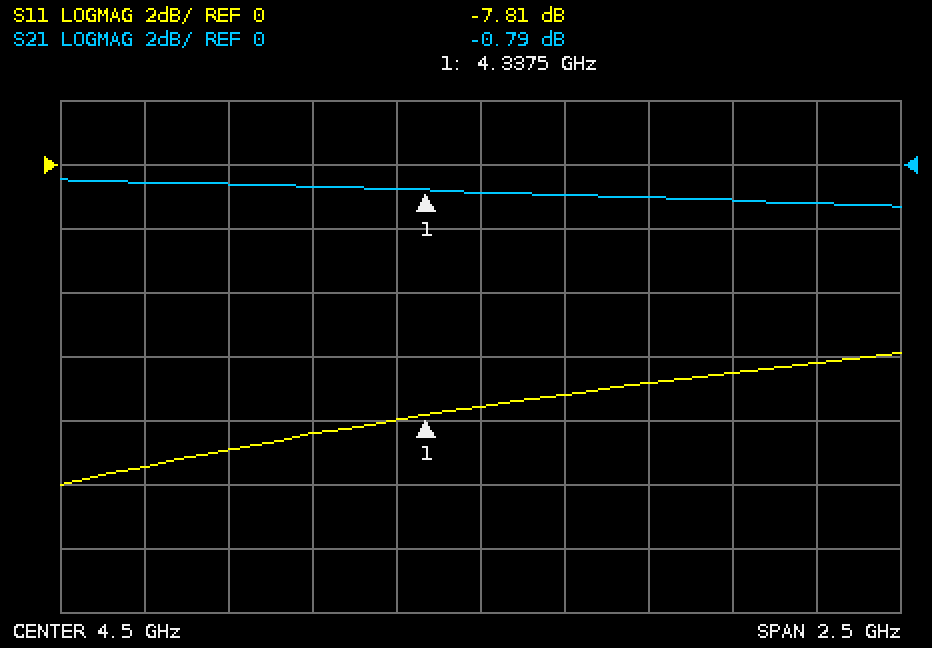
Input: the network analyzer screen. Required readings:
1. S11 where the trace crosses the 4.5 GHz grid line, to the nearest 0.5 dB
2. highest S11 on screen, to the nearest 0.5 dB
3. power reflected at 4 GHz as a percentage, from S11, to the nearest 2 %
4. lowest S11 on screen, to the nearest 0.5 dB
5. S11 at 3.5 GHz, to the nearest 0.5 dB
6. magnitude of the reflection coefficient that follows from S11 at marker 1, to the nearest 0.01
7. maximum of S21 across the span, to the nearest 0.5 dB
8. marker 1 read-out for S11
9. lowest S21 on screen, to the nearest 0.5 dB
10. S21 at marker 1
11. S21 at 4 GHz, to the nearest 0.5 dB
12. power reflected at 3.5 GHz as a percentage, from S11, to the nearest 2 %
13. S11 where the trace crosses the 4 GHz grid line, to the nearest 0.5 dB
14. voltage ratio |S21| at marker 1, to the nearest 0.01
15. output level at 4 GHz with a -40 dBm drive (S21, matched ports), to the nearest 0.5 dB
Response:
-7.5 dB
-6.0 dB
14 %
-10.0 dB
-9.5 dB
0.41
-0.5 dB
-7.81 dB
-1.5 dB
-0.79 dB
-0.5 dB
12 %
-8.5 dB
0.91
-40.5 dBm
